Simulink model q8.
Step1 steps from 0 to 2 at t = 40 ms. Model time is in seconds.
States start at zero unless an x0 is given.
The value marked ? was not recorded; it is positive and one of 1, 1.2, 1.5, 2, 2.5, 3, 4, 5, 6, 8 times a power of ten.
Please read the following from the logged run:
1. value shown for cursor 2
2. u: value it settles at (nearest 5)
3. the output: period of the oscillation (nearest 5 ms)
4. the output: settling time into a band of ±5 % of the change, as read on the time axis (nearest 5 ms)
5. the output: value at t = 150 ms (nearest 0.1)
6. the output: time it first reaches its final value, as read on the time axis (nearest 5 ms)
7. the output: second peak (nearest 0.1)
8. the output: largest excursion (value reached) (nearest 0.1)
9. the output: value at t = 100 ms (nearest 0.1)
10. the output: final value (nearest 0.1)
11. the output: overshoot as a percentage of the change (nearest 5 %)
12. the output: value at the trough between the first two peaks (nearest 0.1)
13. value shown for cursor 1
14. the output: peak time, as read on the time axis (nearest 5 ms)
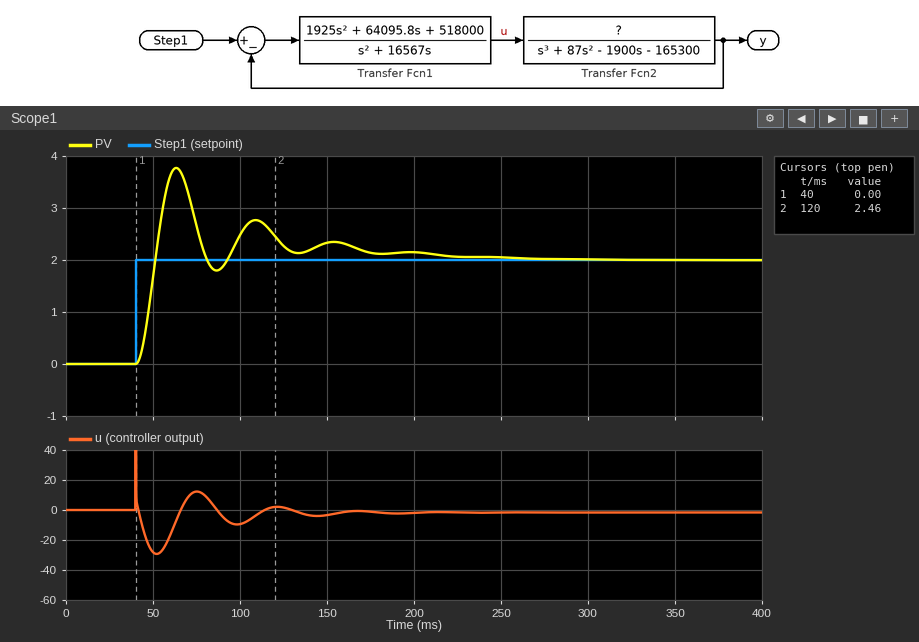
2.46
0
45 ms
215 ms
2.3
50 ms
2.8
3.8
2.5
2.0
90 %
1.8
0.00
65 ms
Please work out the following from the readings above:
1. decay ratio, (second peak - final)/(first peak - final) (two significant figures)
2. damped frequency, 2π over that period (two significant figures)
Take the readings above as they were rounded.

0.44
0.14 rad/ms
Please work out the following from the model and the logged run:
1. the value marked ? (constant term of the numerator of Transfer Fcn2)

200000
